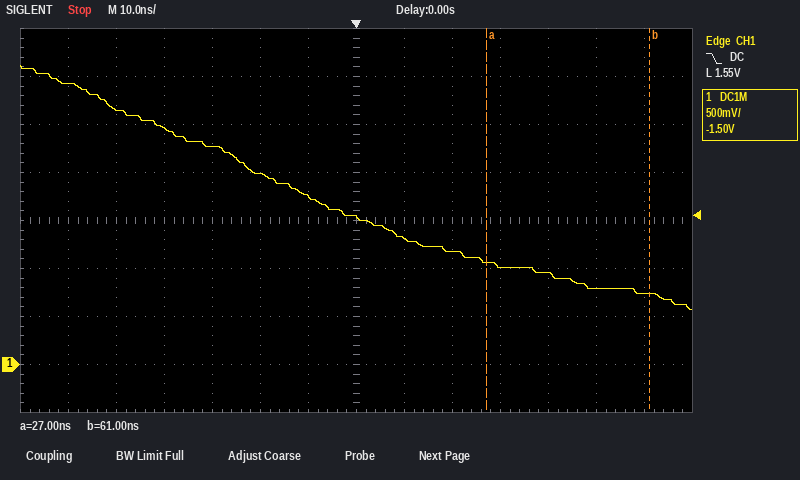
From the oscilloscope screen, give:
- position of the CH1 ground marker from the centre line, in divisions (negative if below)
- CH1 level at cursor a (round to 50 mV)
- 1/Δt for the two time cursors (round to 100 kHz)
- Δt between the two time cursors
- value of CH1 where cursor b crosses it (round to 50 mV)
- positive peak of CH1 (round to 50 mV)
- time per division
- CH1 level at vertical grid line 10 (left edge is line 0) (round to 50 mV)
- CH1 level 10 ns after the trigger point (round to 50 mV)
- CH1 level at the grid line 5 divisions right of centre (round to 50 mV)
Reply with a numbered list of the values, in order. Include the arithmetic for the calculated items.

1. -3.0 div
2. 1.05 V
3. 1 / 34 ns ≈ 29.4 MHz
4. 61 ns − (27 ns) = 34 ns
5. 750 mV
6. 3.10 V
7. 10 ns
8. 1.00 V
9. 1.30 V
10. 800 mV
